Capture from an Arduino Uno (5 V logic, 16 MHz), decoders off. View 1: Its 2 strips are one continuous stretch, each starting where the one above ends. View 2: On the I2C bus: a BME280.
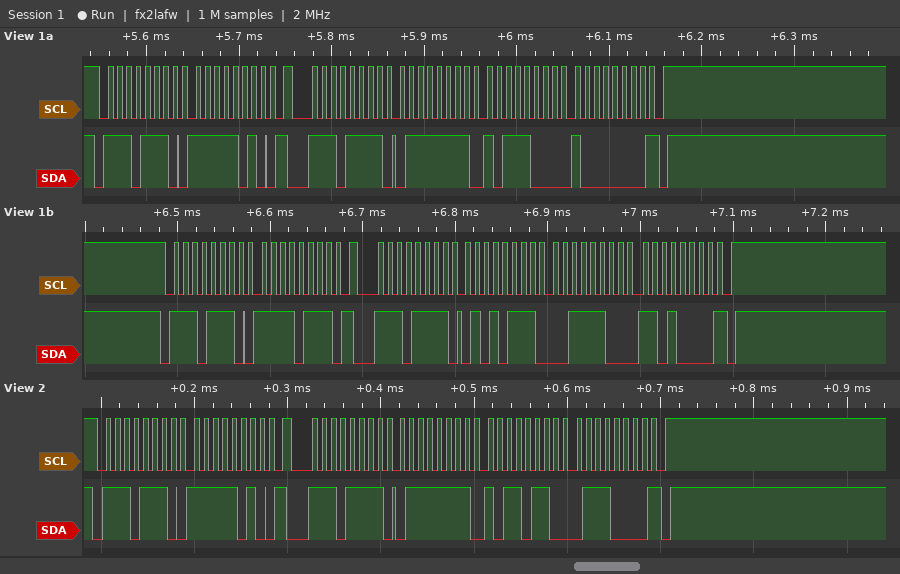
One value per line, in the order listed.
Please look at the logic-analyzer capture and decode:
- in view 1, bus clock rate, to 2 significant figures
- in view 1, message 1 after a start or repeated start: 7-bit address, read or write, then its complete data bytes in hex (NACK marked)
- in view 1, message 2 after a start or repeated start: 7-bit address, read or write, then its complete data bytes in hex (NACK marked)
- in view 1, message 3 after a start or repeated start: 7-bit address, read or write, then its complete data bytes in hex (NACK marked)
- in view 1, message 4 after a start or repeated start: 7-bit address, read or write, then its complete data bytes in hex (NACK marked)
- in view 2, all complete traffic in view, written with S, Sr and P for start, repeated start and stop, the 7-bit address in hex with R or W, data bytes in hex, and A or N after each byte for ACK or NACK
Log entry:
100 kHz
0x77 write: FA
0x77 read: 7F B8 80 NACK
0x77 write: F7
0x77 read: 57 3C D0 NACK
S 77W A FA A Sr 77R A 7F A B6 A 70 N P
